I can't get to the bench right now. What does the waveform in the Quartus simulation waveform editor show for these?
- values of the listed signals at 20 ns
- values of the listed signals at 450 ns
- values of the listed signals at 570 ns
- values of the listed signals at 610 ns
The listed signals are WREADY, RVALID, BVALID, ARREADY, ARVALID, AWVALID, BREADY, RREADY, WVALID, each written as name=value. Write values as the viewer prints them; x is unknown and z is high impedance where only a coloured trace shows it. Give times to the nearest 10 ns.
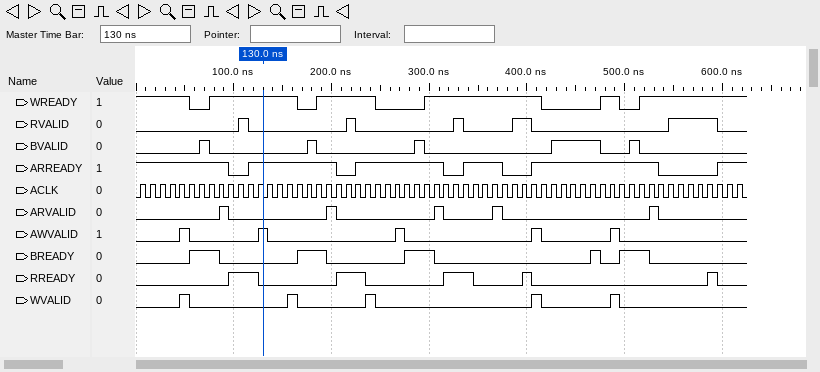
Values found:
WREADY=1, RVALID=0, BVALID=0, ARREADY=1, ARVALID=0, AWVALID=0, BREADY=0, RREADY=0, WVALID=0
WREADY=0, RVALID=0, BVALID=1, ARREADY=1, ARVALID=0, AWVALID=0, BREADY=0, RREADY=0, WVALID=0
WREADY=1, RVALID=1, BVALID=0, ARREADY=0, ARVALID=0, AWVALID=0, BREADY=0, RREADY=0, WVALID=0
WREADY=1, RVALID=0, BVALID=0, ARREADY=1, ARVALID=0, AWVALID=0, BREADY=0, RREADY=0, WVALID=0
